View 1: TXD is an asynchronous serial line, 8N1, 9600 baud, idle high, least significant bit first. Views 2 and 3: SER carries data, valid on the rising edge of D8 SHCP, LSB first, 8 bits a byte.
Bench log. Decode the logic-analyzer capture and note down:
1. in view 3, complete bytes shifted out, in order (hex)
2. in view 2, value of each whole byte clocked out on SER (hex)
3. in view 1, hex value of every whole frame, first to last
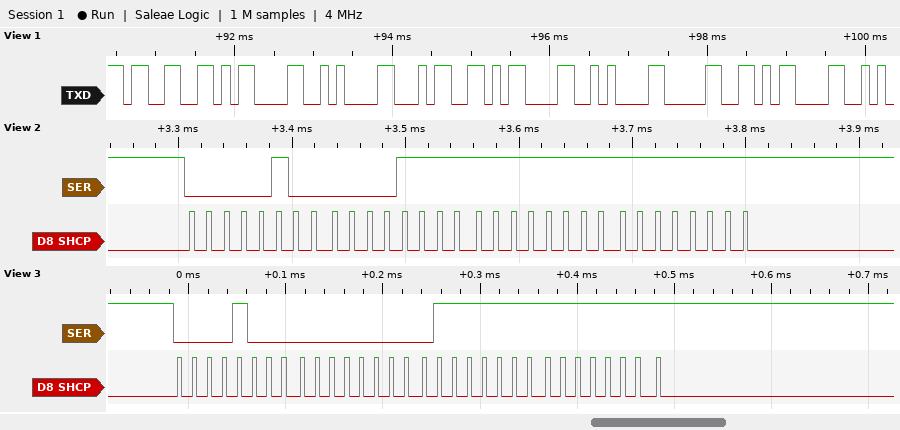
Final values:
0x10 0x00 0xFE 0xFF
20 F0 FF FF
33 0D 0A 34 0D 0A 30 0D
